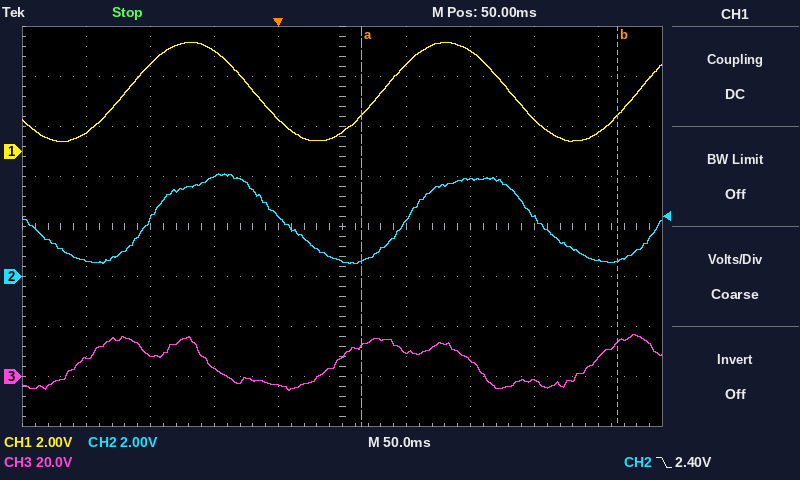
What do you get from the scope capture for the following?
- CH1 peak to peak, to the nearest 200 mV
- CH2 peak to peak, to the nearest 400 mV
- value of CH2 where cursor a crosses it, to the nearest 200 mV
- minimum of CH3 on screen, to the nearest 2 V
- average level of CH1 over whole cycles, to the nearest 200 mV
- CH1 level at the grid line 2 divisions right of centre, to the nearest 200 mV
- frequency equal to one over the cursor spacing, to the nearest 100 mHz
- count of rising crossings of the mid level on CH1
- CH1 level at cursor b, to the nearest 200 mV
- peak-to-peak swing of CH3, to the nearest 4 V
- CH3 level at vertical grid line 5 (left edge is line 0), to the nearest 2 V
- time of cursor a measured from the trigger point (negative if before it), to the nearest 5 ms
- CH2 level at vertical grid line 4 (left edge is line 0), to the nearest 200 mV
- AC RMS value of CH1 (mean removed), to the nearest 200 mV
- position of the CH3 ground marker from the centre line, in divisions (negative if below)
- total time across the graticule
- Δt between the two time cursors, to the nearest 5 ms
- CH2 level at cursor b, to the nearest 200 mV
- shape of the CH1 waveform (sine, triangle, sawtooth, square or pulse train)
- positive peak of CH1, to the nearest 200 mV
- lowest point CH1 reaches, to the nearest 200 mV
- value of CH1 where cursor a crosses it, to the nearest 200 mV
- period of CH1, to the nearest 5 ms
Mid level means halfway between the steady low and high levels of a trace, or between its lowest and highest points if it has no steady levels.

4.0 V
3.6 V
600 mV
-6 V
2.4 V
4.0 V
5.0 Hz
3
1.4 V
24 V
8 V
+65 ms
2.4 V
1.4 V
-3.0 div
500 ms
200 ms
600 mV
sine
4.4 V
400 mV
1.4 V
200 ms
